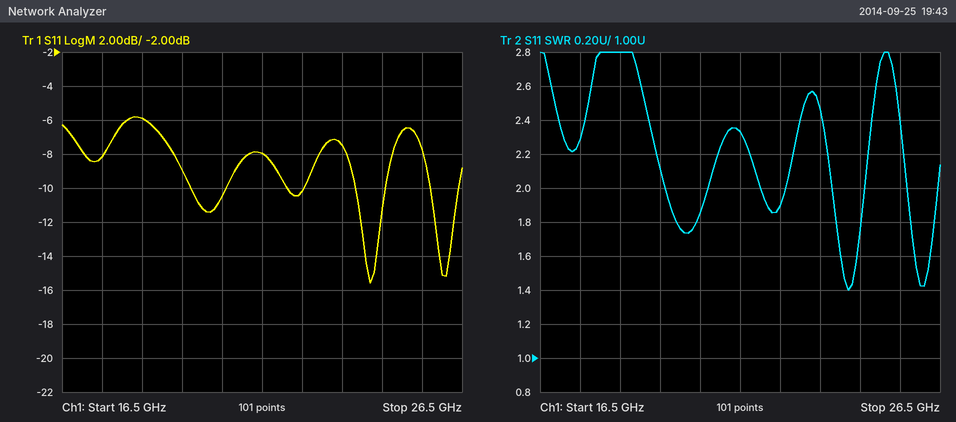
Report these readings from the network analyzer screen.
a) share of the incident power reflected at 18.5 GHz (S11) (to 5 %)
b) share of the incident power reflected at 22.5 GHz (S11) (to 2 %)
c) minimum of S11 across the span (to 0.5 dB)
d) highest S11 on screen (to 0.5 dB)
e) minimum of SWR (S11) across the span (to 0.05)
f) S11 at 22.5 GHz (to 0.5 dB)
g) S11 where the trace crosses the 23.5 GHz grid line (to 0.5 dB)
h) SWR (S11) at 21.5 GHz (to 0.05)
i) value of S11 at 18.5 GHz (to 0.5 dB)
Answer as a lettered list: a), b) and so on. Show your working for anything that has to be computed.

a) 10^(-6/10) ≈ 25 %
b) 10^(-10/10) ≈ 10 %
c) -15.5 dB
d) -6.0 dB
e) 1.40
f) -10.0 dB
g) -7.5 dB
h) 2.35
i) -6.0 dB
